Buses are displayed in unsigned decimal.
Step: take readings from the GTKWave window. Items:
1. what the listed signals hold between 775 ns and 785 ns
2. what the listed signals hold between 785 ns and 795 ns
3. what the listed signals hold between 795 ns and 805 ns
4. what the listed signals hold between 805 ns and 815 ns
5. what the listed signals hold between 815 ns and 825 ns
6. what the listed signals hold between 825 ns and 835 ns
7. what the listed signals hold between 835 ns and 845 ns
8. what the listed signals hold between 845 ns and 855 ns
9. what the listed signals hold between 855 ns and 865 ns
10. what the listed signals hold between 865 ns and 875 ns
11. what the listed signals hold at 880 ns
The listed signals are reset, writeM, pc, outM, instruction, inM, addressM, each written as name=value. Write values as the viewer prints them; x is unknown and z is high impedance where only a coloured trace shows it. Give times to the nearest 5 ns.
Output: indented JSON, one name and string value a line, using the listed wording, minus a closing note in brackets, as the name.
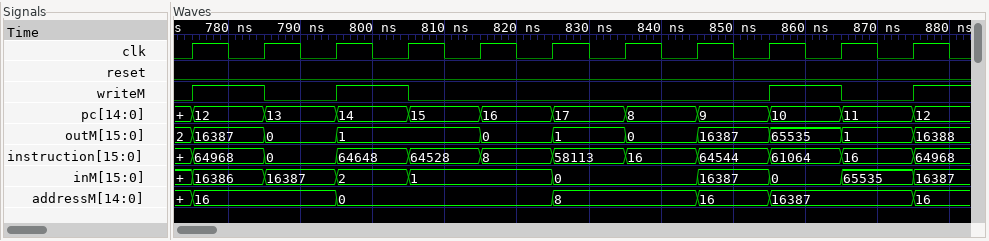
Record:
{
  "what the listed signals hold between 775 ns and 785 ns": "reset=0, writeM=1, pc=12, outM=16387, instruction=64968, inM=16386, addressM=16",
  "what the listed signals hold between 785 ns and 795 ns": "reset=0, writeM=0, pc=13, outM=0, instruction=0, inM=16387, addressM=16",
  "what the listed signals hold between 795 ns and 805 ns": "reset=0, writeM=1, pc=14, outM=1, instruction=64648, inM=2, addressM=0",
  "what the listed signals hold between 805 ns and 815 ns": "reset=0, writeM=0, pc=15, outM=1, instruction=64528, inM=1, addressM=0",
  "what the listed signals hold between 815 ns and 825 ns": "reset=0, writeM=0, pc=16, outM=0, instruction=8, inM=1, addressM=0",
  "what the listed signals hold between 825 ns and 835 ns": "reset=0, writeM=0, pc=17, outM=1, instruction=58113, inM=0, addressM=8",
  "what the listed signals hold between 835 ns and 845 ns": "reset=0, writeM=0, pc=8, outM=0, instruction=16, inM=0, addressM=8",
  "what the listed signals hold between 845 ns and 855 ns": "reset=0, writeM=0, pc=9, outM=16387, instruction=64544, inM=16387, addressM=16",
  "what the listed signals hold between 855 ns and 865 ns": "reset=0, writeM=1, pc=10, outM=65535, instruction=61064, inM=0, addressM=16387",
  "what the listed signals hold between 865 ns and 875 ns": "reset=0, writeM=0, pc=11, outM=1, instruction=16, inM=65535, addressM=16387",
  "what the listed signals hold at 880 ns": "reset=0, writeM=1, pc=12, outM=16388, instruction=64968, inM=16387, addressM=16"
}
